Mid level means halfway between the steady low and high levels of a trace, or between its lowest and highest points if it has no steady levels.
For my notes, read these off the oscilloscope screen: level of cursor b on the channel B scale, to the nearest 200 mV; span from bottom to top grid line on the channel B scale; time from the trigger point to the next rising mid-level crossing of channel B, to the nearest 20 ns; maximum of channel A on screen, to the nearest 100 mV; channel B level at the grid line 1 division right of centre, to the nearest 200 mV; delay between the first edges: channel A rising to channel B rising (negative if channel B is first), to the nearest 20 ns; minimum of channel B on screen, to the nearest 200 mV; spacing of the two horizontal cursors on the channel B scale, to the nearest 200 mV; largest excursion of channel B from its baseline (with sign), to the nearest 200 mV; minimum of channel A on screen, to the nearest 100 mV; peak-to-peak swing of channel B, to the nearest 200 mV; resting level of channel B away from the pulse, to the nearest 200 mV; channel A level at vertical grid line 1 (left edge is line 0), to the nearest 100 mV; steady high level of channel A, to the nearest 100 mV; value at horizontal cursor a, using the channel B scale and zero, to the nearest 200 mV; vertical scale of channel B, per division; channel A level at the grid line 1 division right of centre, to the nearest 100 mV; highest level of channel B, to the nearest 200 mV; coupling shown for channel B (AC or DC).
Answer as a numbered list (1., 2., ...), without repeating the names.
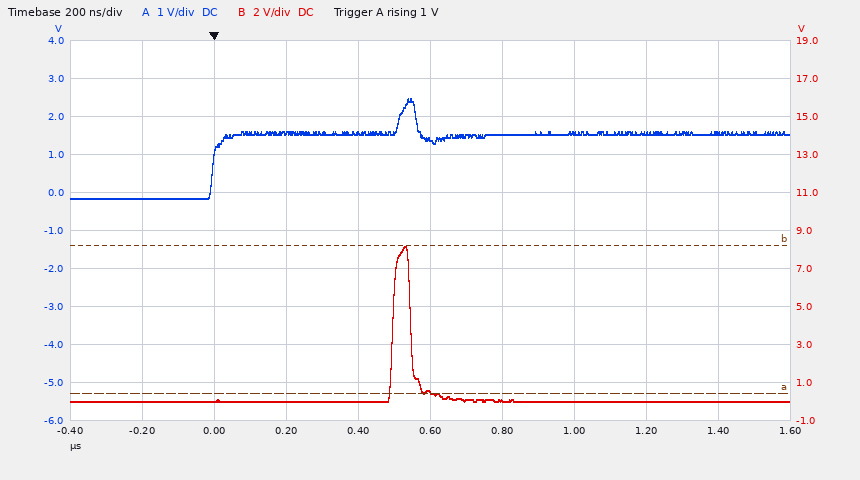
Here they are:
1. 8.2 V
2. 20 V
3. 500 ns
4. 2.5 V
5. 0.0 V
6. +500 ns
7. 0.0 V
8. 7.8 V
9. +8.2 V
10. -200 mV
11. 8.2 V
12. 0.0 V
13. -200 mV
14. 1.5 V
15. 400 mV
16. 2 V
17. 1.5 V
18. 8.2 V
19. DC
